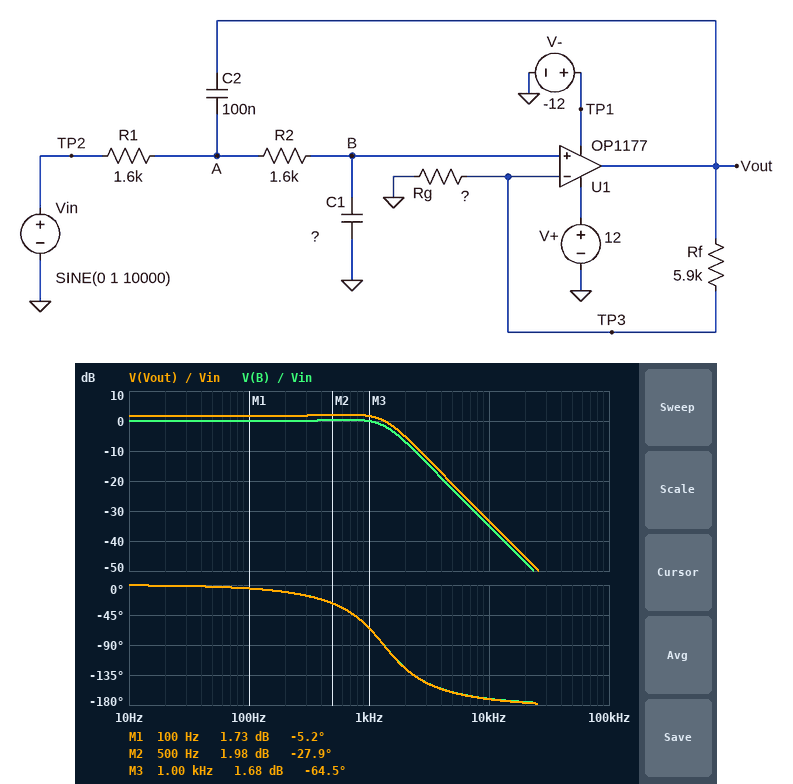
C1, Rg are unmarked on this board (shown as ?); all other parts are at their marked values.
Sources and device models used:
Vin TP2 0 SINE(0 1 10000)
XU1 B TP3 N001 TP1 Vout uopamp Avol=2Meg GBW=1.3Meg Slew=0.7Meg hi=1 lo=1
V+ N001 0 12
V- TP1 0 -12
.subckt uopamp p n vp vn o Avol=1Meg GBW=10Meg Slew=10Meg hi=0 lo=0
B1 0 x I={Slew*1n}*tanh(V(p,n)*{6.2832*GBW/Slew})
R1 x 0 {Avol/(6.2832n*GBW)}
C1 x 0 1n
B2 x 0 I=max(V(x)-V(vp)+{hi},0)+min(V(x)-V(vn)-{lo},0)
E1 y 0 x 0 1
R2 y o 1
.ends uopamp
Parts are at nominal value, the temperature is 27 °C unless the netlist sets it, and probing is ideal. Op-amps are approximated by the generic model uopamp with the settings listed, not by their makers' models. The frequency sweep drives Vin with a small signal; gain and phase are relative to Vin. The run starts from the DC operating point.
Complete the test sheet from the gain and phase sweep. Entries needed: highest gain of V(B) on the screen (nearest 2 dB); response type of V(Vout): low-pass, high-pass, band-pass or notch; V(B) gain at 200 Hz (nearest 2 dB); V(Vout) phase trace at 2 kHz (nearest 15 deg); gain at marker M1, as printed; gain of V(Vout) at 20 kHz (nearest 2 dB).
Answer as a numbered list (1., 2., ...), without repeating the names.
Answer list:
1. 0 dB
2. low-pass
3. 0 dB
4. -120 deg
5. 1.73 dB
6. -46 dB
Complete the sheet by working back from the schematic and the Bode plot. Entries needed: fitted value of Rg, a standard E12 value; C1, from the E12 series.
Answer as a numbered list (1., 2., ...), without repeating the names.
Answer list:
1. 27 kΩ
2. 56 nF
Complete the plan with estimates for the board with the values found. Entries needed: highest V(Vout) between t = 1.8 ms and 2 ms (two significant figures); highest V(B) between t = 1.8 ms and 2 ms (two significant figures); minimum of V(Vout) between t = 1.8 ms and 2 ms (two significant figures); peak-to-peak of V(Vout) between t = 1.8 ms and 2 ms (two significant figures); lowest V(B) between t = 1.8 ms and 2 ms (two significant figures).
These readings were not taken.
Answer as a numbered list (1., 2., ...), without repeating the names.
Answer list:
1. 22 mV
2. 18 mV
3. -22 mV
4. 43 mV
5. -18 mV
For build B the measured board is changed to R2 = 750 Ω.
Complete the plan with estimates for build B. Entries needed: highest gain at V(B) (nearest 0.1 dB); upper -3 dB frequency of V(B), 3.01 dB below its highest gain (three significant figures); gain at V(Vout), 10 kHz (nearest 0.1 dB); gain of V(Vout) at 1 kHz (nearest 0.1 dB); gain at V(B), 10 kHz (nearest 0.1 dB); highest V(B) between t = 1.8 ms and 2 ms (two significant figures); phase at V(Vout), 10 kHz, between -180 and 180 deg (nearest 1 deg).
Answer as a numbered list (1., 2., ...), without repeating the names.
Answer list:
1. 0.4 dB
2. 2.17 kHz
3. -26.7 dB
4. 2.1 dB
5. -28.4 dB
6. 38 mV
7. -167 deg
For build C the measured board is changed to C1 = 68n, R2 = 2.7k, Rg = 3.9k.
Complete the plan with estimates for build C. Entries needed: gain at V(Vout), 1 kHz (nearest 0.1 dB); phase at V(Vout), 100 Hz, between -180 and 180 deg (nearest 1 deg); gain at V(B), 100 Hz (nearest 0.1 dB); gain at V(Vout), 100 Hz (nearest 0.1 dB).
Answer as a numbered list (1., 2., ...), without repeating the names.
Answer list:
1. 17.0 dB
2. -2 deg
3. 0.1 dB
4. 8.1 dB
